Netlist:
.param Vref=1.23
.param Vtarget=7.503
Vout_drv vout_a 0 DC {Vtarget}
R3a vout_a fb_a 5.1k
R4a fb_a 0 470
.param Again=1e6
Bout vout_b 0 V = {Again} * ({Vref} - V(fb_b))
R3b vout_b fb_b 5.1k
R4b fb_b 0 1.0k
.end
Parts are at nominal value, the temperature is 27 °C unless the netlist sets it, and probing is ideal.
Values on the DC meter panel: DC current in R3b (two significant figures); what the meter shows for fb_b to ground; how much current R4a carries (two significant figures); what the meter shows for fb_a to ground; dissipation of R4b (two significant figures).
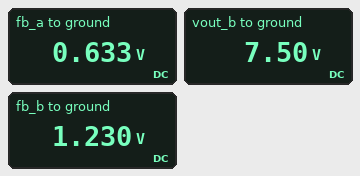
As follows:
1.2 mA
1.230 V
1.3 mA
0.633 V
1.5 mW
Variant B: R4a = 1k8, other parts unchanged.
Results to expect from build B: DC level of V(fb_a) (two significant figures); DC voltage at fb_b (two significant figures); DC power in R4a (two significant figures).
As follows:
2.0 V
1.2 V
2.1 mW
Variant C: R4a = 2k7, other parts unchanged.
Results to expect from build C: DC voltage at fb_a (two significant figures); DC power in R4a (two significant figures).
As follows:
2.6 V
2.5 mW
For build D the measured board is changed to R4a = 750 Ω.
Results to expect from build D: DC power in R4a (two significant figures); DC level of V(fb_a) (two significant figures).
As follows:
1.2 mW
960 mV
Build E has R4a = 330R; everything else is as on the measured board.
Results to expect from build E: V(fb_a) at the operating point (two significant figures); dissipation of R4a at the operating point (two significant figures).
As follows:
460 mV
630 µW
